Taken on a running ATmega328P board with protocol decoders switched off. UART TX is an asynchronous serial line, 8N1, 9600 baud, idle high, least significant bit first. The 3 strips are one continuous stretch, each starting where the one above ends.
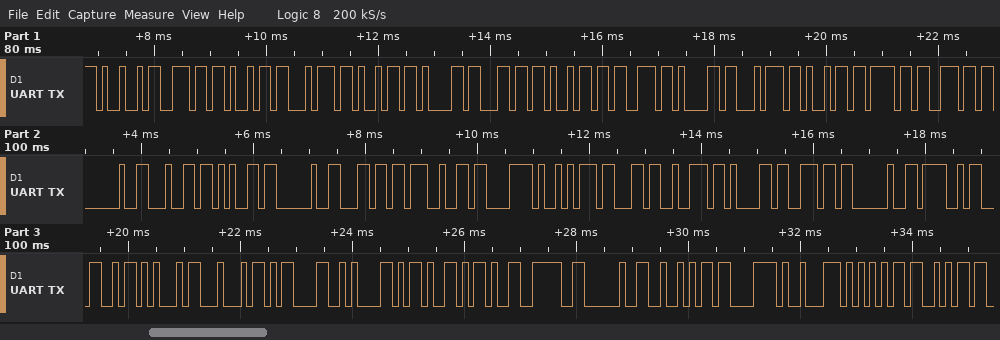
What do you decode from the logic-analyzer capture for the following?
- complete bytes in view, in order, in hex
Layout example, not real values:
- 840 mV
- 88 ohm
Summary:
- 49 6E 69 74 69 61 6C 69 73 61 74 69 6F 6E 20 64 65 20 6C 27 C3 A9 63 72 61 6E 20 4F 4C 45 44 0D 0A 2D 2D 3E 20 52 C3 89 55 53
